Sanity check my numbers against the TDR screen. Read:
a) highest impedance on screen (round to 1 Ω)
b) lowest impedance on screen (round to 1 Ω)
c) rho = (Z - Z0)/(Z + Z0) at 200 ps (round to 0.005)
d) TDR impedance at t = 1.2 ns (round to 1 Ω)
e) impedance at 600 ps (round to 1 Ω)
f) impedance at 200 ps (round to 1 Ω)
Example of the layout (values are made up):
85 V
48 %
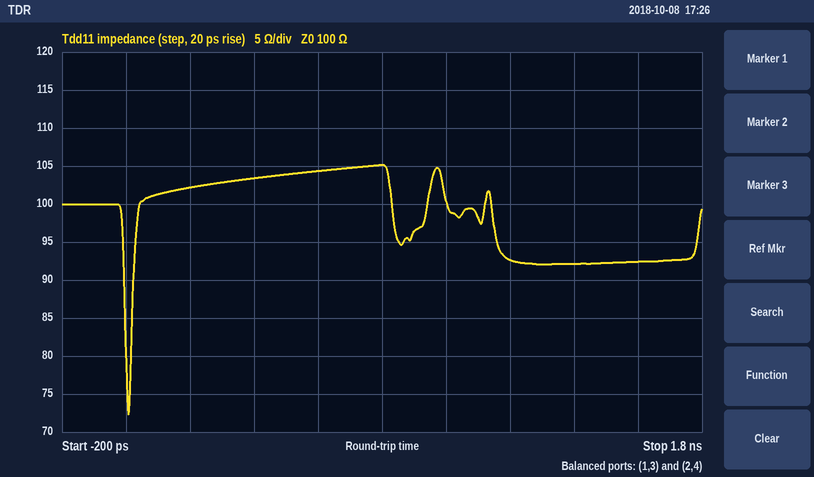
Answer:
105 Ω
72 Ω
+0.010
93 Ω
104 Ω
102 Ω
